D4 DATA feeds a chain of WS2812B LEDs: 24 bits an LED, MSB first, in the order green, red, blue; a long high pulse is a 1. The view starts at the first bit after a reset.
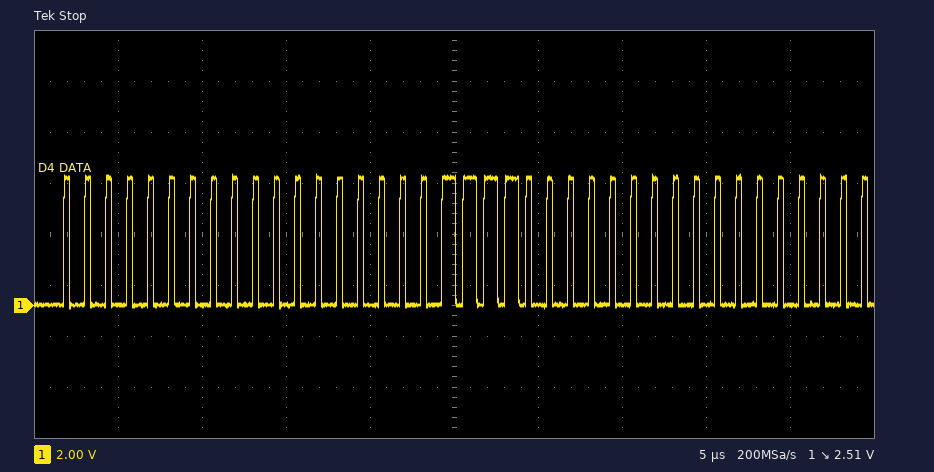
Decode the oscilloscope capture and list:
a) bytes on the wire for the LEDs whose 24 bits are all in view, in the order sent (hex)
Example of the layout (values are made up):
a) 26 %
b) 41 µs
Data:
a) 00 00 3C
